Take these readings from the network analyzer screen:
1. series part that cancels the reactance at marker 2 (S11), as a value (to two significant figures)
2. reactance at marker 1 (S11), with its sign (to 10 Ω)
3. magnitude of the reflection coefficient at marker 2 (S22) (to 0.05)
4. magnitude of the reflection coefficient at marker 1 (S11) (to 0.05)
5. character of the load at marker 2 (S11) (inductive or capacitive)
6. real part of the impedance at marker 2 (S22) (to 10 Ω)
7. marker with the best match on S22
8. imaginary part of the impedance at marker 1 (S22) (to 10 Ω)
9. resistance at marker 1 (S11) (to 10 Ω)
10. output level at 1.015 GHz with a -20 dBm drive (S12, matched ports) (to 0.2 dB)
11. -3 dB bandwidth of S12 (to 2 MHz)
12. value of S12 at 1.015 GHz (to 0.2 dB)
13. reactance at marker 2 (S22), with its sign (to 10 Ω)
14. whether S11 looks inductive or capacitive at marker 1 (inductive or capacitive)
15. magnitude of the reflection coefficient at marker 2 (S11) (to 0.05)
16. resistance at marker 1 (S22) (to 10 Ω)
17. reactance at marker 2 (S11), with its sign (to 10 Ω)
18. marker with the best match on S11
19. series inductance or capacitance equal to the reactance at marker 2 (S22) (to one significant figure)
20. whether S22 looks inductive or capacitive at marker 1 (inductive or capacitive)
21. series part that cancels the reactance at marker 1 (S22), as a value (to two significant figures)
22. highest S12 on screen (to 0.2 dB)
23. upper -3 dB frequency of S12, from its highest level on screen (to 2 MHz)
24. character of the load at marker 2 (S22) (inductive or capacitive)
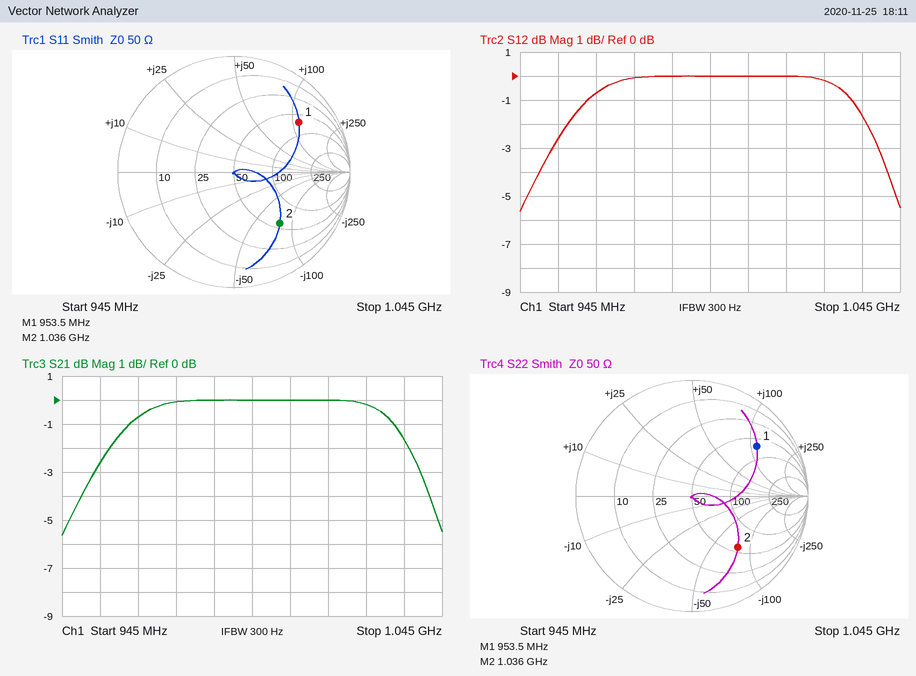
12 nH
+110 Ω
0.60
0.70
capacitive
60 Ω
marker 2
+110 Ω
70 Ω
-20.0 dBm
86 MHz
0.0 dB
-80 Ω
inductive
0.60
70 Ω
-80 Ω
marker 2
2 pF
inductive
1.5 pF
0.0 dB
1.040 GHz
capacitive
